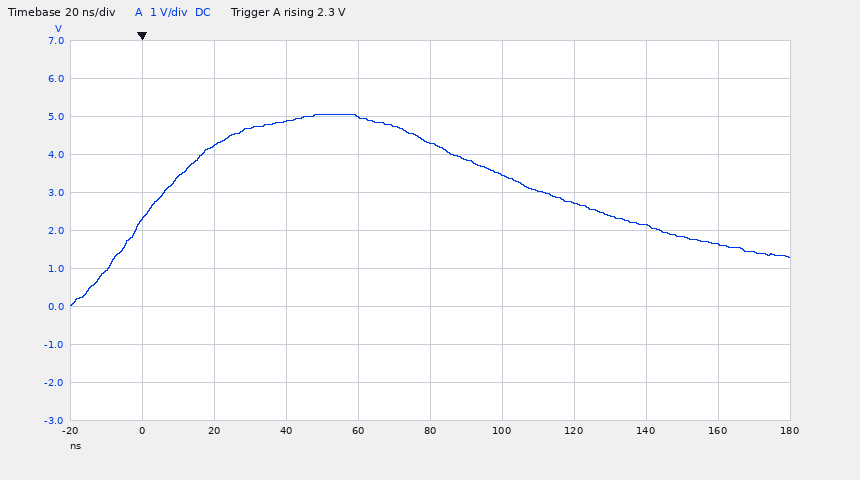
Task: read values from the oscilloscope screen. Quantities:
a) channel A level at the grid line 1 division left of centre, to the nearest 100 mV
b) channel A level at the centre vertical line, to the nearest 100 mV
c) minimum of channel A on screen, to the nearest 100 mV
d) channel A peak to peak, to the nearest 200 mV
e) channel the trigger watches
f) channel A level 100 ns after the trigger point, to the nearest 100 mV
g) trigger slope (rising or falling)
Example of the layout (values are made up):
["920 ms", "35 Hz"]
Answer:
["5.0 V", "4.3 V", "0.0 V", "5.0 V", "channel A", "3.5 V", "rising"]
